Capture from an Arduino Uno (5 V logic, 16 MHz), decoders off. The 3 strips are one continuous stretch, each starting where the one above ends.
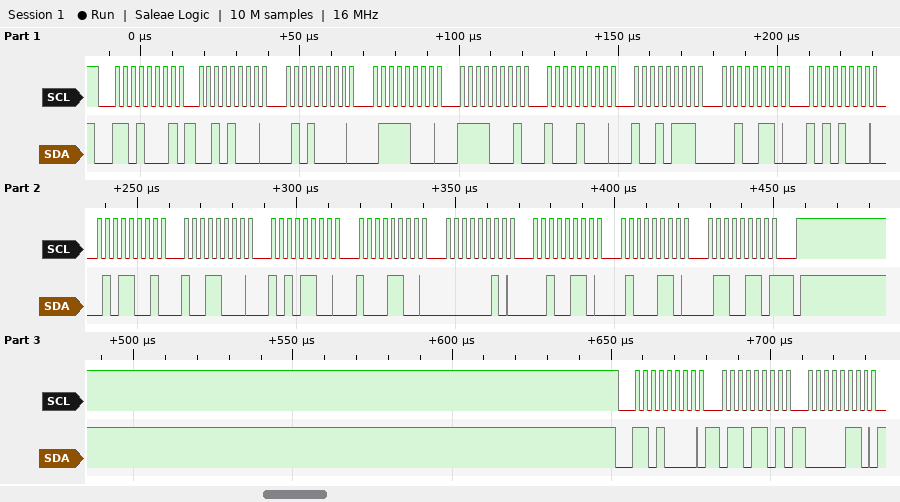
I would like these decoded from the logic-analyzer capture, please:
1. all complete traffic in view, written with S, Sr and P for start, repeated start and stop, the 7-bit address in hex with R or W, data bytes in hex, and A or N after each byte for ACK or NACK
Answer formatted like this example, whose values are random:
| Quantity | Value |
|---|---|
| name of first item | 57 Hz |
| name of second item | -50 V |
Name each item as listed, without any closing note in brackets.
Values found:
| Quantity | Value |
|---|---|
| all complete traffic in view, written with S, Sr and P for start, repeated start and stop, the 7-bit address in hex with R or W, data bytes in hex, and A or N after each byte for ACK or NACK | S 68R A 28 A 50 A 78 A F1 A 88 A 97 A 26 A A8 A 59 A 98 A AC A 8C A 02 A 26 A 46 A 66 N P S 68W A 6D A 06 A |
